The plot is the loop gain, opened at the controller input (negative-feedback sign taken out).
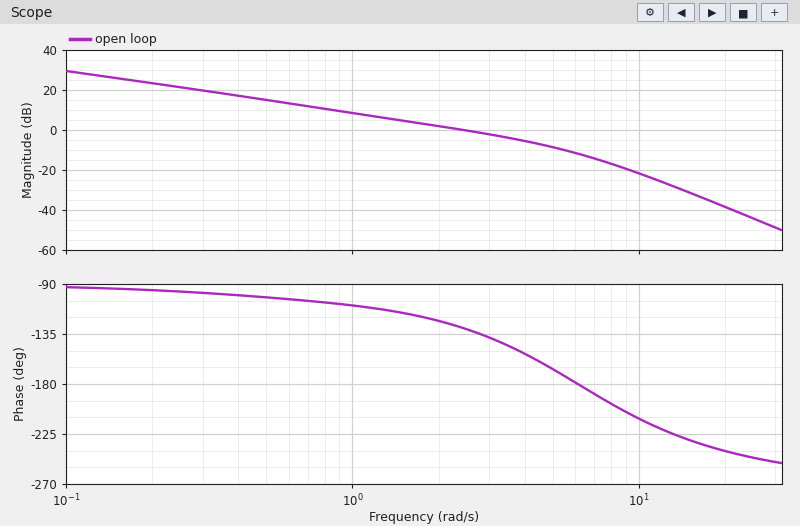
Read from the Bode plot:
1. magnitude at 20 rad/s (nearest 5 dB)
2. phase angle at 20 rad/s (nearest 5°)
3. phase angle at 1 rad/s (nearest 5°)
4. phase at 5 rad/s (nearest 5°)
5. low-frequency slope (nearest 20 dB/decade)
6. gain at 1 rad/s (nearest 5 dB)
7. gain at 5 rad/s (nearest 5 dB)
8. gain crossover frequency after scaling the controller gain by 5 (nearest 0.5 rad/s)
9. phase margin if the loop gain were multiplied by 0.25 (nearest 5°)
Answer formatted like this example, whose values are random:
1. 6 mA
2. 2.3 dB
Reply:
1. -40 dB
2. -240°
3. -110°
4. -165°
5. -20 dB/decade
6. 10 dB
7. -10 dB
8. 7.0 rad/s
9. 75°
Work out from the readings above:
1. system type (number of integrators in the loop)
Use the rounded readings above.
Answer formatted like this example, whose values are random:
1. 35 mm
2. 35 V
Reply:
1. 1
